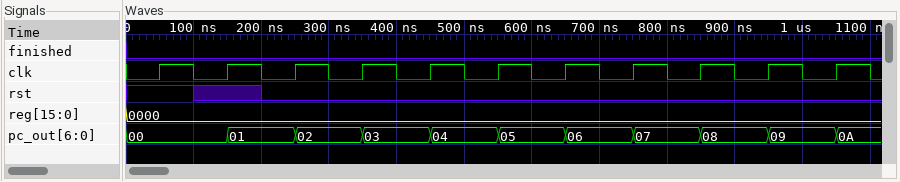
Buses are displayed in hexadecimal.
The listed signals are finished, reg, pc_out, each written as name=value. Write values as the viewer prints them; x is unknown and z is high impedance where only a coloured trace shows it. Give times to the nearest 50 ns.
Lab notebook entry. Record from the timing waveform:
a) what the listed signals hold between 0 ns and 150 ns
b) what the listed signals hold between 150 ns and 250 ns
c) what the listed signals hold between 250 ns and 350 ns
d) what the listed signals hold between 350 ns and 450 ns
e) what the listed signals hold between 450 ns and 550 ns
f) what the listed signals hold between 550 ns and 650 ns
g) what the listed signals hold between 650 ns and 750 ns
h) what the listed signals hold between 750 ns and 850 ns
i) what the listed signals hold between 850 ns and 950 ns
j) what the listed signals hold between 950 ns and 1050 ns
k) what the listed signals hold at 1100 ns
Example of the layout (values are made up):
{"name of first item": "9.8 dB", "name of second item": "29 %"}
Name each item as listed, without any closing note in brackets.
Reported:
{"what the listed signals hold between 0 ns and 150 ns": "finished=0, reg=0000, pc_out=00", "what the listed signals hold between 150 ns and 250 ns": "finished=0, reg=0000, pc_out=01", "what the listed signals hold between 250 ns and 350 ns": "finished=0, reg=0000, pc_out=02", "what the listed signals hold between 350 ns and 450 ns": "finished=0, reg=0000, pc_out=03", "what the listed signals hold between 450 ns and 550 ns": "finished=0, reg=0000, pc_out=04", "what the listed signals hold between 550 ns and 650 ns": "finished=0, reg=0000, pc_out=05", "what the listed signals hold between 650 ns and 750 ns": "finished=0, reg=0000, pc_out=06", "what the listed signals hold between 750 ns and 850 ns": "finished=0, reg=0000, pc_out=07", "what the listed signals hold between 850 ns and 950 ns": "finished=0, reg=0000, pc_out=08", "what the listed signals hold between 950 ns and 1050 ns": "finished=0, reg=0000, pc_out=09", "what the listed signals hold at 1100 ns": "finished=0, reg=0000, pc_out=0A"}
